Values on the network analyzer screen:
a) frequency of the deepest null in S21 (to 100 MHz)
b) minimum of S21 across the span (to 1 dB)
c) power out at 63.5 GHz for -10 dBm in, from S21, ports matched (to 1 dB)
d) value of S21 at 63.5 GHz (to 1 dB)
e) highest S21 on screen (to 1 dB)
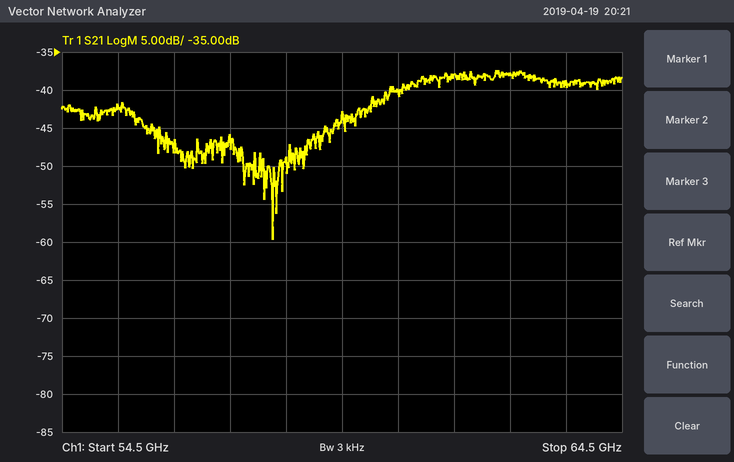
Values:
58.3 GHz
-60 dB
-49 dBm
-39 dB
-37 dB
